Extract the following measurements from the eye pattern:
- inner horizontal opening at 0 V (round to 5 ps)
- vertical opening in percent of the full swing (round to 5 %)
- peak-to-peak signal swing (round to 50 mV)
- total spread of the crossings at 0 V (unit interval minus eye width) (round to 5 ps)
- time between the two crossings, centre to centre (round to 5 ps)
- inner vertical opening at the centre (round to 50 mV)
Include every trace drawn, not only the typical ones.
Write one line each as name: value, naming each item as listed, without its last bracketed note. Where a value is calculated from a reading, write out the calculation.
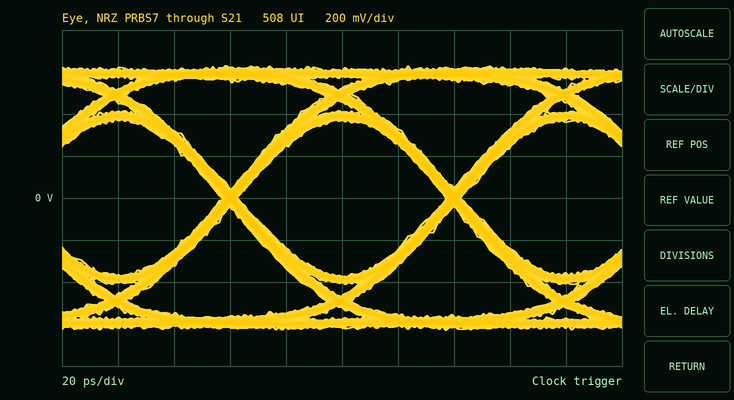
inner horizontal opening at 0 V: 75 ps
vertical opening in percent of the full swing: 750 mV / 1.25 V ≈ 60 %
peak-to-peak signal swing: 1.25 V
total spread of the crossings at 0 V (unit interval minus eye width): 5 ps
time between the two crossings, centre to centre: 80 ps
inner vertical opening at the centre: 750 mV
